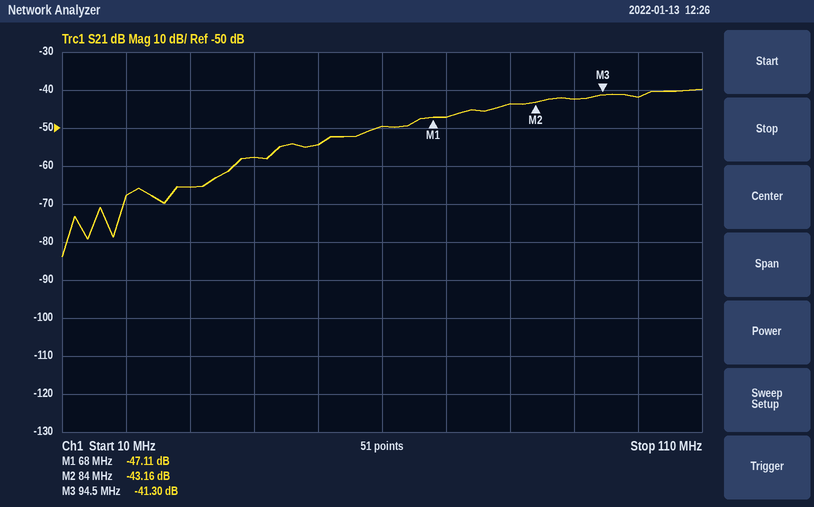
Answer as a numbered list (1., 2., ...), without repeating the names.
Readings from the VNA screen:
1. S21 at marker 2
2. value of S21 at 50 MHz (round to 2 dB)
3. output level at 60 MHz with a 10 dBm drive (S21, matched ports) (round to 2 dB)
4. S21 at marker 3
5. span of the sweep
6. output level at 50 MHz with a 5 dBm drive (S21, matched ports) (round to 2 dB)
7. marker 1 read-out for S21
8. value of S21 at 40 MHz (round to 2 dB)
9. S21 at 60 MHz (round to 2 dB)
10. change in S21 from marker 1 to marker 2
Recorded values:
1. -43.16 dB
2. -54 dB
3. -40 dBm
4. -41.30 dB
5. 100 MHz
6. -50 dBm
7. -47.11 dB
8. -58 dB
9. -50 dB
10. 3.95 dB
